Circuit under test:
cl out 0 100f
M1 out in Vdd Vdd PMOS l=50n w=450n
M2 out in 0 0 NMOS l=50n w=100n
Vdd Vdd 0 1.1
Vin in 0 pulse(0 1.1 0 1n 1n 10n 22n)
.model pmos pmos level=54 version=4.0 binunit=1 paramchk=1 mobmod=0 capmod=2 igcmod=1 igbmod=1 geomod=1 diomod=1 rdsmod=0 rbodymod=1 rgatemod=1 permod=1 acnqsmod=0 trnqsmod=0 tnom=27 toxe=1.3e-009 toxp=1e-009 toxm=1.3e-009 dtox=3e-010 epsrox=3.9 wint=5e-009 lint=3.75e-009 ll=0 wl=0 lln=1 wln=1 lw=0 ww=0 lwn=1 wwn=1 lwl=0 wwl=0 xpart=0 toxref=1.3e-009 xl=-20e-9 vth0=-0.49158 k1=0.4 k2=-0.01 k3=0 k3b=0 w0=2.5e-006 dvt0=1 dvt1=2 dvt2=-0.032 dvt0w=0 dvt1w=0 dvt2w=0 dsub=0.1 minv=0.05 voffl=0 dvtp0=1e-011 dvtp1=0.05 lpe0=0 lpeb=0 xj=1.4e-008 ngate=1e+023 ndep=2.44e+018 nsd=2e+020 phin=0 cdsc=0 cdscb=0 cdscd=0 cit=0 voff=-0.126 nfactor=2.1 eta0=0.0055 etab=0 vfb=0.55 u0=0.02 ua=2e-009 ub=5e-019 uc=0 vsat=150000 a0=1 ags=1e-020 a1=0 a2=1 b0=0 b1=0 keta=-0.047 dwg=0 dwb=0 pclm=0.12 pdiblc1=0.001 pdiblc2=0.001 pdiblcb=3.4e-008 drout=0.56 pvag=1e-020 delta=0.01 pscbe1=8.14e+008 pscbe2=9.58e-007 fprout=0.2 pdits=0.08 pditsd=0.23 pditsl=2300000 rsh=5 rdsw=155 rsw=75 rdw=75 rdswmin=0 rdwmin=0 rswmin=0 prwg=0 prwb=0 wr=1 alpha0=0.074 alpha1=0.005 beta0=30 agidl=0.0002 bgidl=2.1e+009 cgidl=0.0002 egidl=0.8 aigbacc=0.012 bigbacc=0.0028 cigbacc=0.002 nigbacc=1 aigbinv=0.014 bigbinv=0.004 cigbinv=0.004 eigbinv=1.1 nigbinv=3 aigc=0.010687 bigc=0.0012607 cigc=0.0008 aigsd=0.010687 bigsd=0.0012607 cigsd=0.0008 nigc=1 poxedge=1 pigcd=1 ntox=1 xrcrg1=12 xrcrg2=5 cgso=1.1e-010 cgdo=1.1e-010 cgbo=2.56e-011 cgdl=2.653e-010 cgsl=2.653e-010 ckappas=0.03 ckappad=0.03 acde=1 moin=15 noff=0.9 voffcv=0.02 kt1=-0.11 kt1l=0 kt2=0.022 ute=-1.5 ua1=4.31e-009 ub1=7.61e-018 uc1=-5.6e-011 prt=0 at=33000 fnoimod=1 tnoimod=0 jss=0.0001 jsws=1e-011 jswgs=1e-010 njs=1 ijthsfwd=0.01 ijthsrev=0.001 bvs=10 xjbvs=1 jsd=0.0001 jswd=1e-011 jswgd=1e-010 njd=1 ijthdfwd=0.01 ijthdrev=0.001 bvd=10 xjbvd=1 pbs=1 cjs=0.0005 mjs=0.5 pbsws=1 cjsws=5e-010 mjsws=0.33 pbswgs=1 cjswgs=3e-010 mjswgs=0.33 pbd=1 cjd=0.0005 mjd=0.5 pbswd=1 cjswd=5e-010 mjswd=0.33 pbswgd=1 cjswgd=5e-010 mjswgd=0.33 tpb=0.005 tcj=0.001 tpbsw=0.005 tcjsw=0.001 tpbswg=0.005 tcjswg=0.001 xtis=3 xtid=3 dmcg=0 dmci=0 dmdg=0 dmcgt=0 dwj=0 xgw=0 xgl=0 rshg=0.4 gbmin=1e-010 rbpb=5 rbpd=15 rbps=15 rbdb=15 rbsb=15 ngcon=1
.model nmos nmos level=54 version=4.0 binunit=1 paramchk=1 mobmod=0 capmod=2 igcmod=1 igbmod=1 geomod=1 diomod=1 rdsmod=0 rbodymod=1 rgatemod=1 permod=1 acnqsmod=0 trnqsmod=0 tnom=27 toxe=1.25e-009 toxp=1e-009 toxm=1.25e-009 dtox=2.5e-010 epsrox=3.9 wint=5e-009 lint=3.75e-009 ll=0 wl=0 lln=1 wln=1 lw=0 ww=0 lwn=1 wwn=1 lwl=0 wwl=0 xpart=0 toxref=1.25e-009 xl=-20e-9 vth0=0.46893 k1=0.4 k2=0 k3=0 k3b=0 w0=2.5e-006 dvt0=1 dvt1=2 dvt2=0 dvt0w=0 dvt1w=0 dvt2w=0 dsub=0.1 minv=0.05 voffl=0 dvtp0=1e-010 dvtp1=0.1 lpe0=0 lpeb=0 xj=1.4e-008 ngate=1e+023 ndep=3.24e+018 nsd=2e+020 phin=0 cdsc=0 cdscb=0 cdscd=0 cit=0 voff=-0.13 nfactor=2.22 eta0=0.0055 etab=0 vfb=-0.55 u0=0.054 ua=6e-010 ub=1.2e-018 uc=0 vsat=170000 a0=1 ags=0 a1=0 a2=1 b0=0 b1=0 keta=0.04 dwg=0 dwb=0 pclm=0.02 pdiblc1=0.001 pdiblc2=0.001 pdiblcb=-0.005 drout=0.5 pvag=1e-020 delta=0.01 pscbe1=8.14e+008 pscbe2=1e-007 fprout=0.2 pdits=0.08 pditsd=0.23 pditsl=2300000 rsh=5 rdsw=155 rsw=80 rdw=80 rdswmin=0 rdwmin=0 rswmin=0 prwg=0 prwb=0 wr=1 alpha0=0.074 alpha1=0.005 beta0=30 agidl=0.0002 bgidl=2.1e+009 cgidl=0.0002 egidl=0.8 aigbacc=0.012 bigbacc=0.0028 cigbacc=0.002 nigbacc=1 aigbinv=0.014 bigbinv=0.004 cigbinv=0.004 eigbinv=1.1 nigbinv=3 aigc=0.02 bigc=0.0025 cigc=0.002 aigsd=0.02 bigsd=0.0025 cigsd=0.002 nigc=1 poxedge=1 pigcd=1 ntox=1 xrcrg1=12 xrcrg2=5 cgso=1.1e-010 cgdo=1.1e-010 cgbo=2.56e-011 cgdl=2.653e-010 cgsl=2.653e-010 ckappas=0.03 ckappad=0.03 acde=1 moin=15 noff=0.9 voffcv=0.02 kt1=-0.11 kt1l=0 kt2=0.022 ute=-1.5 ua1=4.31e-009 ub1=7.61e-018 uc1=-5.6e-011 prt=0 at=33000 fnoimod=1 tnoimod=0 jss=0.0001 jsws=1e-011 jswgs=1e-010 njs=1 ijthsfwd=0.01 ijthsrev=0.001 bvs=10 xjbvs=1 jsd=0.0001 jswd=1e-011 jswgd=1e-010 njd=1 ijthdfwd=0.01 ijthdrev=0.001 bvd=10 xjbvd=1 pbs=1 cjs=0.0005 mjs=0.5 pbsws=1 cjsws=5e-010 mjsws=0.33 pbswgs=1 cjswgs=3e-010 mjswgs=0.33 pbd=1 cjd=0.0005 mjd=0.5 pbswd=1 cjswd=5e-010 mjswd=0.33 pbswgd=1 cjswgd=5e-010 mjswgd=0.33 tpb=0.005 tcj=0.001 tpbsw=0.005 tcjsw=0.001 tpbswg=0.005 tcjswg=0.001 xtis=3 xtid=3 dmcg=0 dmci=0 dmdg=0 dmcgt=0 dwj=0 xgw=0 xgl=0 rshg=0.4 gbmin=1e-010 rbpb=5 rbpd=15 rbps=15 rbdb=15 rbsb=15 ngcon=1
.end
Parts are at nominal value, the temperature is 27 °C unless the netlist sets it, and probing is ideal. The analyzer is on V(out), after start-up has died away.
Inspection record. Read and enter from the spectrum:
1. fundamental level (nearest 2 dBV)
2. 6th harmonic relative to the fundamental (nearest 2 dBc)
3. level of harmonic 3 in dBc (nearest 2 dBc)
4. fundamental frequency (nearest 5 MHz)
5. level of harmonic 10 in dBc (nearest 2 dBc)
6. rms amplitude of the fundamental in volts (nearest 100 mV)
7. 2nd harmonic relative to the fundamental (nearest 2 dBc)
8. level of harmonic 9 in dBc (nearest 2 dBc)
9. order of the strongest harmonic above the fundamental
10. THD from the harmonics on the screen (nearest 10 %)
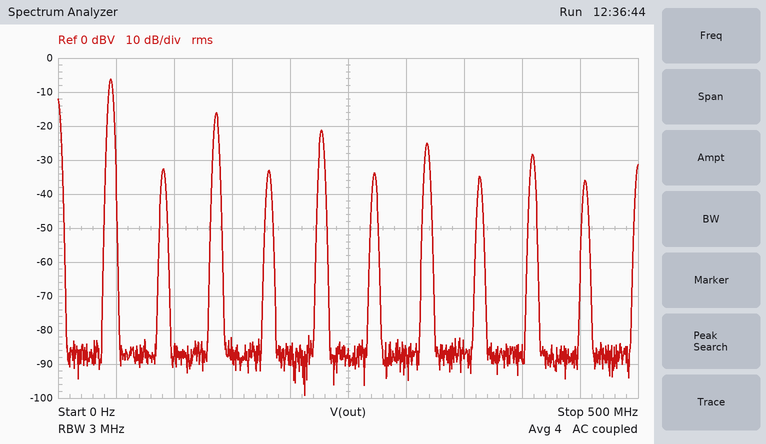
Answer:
-6 dBV
-28 dBc
-10 dBc
45 MHz
-30 dBc
500 mV
-26 dBc
-22 dBc
3
40 %
